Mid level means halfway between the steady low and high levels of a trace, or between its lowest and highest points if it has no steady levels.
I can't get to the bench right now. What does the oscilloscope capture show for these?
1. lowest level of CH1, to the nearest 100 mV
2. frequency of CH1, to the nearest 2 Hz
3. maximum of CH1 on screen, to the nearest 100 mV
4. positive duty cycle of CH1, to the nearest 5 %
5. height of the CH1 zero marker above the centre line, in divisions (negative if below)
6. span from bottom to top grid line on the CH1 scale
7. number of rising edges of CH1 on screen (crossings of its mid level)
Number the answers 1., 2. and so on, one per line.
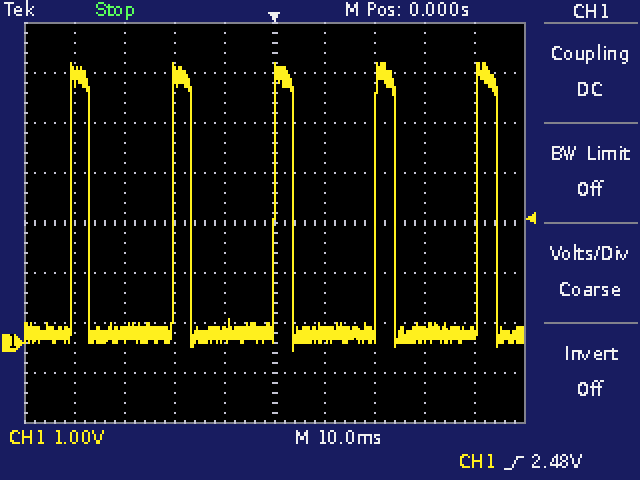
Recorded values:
1. -200 mV
2. 50 Hz
3. 5.6 V
4. 20 %
5. -2.4 div
6. 8 V
7. 5
